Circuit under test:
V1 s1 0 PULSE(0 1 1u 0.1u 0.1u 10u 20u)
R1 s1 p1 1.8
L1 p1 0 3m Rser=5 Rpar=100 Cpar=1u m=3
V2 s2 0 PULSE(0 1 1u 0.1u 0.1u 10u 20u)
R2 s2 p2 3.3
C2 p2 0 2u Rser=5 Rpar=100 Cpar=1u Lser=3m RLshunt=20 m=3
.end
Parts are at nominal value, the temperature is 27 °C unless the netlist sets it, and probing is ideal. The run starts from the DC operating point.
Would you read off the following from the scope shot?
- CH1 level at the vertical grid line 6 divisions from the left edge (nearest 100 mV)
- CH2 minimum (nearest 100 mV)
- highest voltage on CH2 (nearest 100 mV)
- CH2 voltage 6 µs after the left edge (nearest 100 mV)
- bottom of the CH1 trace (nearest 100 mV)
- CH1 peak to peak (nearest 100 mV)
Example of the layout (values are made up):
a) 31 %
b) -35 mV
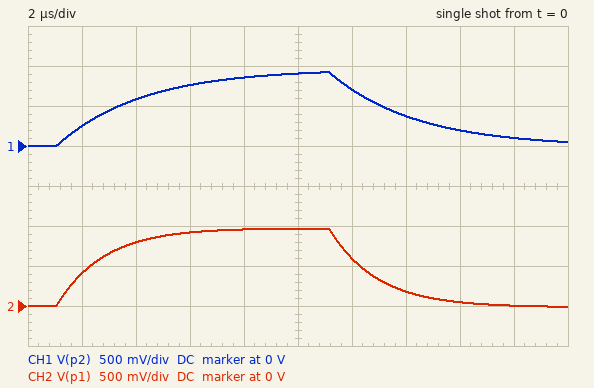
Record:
a) 700 mV
b) 0 V
c) 1.0 V
d) 900 mV
e) 0 V
f) 900 mV
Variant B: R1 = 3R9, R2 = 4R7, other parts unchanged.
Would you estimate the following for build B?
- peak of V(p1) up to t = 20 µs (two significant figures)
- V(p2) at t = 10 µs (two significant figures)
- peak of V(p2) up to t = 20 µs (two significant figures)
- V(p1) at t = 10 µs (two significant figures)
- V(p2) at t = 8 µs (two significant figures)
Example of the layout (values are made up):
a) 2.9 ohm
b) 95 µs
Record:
a) 880 mV
b) 820 mV
c) 850 mV
d) 860 mV
e) 750 mV
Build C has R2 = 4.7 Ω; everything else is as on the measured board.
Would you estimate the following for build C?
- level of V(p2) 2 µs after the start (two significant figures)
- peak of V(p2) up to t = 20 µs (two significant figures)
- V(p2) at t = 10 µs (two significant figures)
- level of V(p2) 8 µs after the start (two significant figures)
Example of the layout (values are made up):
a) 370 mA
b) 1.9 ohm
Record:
a) 180 mV
b) 850 mV
c) 820 mV
d) 750 mV
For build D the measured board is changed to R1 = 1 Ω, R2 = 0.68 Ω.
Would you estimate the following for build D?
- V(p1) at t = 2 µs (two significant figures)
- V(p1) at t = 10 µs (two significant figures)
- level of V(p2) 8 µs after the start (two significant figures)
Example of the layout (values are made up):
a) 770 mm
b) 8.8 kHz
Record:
a) 610 mV
b) 980 mV
c) 990 mV
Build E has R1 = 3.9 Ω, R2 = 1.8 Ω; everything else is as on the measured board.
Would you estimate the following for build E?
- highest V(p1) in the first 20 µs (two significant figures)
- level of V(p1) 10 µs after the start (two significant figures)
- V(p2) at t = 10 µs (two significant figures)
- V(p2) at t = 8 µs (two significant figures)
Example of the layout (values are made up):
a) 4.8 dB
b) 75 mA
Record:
a) 880 mV
b) 860 mV
c) 970 mV
d) 960 mV
